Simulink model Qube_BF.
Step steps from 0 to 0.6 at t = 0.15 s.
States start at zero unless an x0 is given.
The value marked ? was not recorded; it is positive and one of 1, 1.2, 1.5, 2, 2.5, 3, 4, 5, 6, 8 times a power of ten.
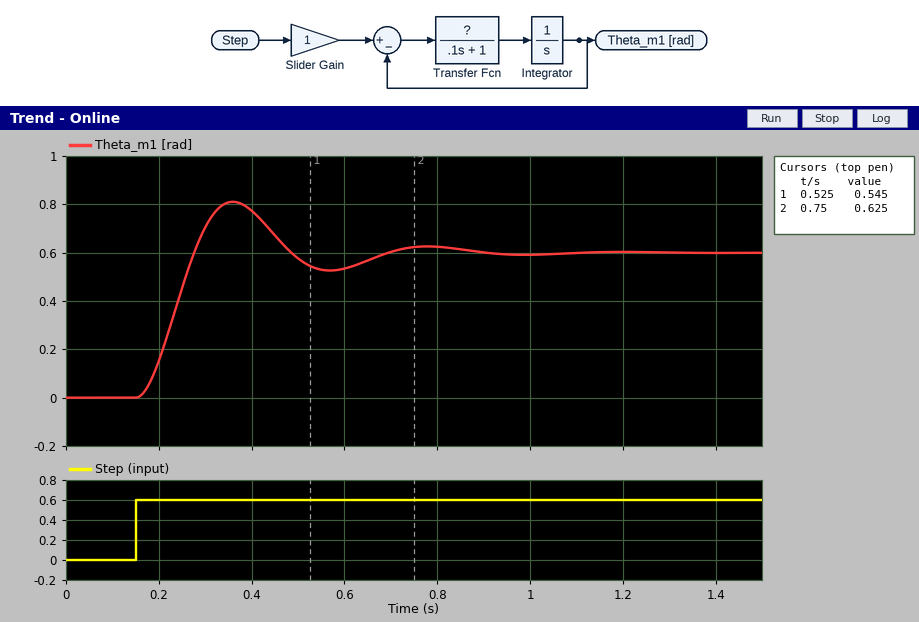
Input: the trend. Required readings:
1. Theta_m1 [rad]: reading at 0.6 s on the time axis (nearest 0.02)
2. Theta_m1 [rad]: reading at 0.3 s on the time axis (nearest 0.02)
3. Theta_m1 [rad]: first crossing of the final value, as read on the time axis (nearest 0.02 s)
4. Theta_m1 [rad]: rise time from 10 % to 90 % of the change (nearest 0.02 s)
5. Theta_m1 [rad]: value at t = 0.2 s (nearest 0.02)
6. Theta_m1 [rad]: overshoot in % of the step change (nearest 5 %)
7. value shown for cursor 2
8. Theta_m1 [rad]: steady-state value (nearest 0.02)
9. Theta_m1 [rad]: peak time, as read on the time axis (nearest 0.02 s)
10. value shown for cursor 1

0.54
0.70
0.28 s
0.08 s
0.16
35 %
0.625
0.60
0.36 s
0.545
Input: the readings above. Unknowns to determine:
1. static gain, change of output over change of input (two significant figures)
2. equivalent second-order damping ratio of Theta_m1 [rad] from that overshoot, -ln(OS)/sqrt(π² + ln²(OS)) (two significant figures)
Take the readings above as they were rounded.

1.0
0.32
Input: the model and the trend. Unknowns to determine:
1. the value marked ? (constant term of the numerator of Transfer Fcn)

25
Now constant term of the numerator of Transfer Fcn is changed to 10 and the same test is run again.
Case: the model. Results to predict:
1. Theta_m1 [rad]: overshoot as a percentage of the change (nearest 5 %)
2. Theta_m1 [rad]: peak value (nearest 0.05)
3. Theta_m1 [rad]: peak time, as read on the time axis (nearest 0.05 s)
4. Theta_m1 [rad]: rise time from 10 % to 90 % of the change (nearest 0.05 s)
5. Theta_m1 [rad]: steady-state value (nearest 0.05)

15 %
0.70
0.50 s
0.15 s
0.60
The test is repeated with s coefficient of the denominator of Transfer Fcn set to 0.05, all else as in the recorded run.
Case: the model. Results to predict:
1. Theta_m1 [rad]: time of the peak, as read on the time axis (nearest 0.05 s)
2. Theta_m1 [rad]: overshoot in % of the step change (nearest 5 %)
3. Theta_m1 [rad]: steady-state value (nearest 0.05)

0.30 s
20 %
0.60
